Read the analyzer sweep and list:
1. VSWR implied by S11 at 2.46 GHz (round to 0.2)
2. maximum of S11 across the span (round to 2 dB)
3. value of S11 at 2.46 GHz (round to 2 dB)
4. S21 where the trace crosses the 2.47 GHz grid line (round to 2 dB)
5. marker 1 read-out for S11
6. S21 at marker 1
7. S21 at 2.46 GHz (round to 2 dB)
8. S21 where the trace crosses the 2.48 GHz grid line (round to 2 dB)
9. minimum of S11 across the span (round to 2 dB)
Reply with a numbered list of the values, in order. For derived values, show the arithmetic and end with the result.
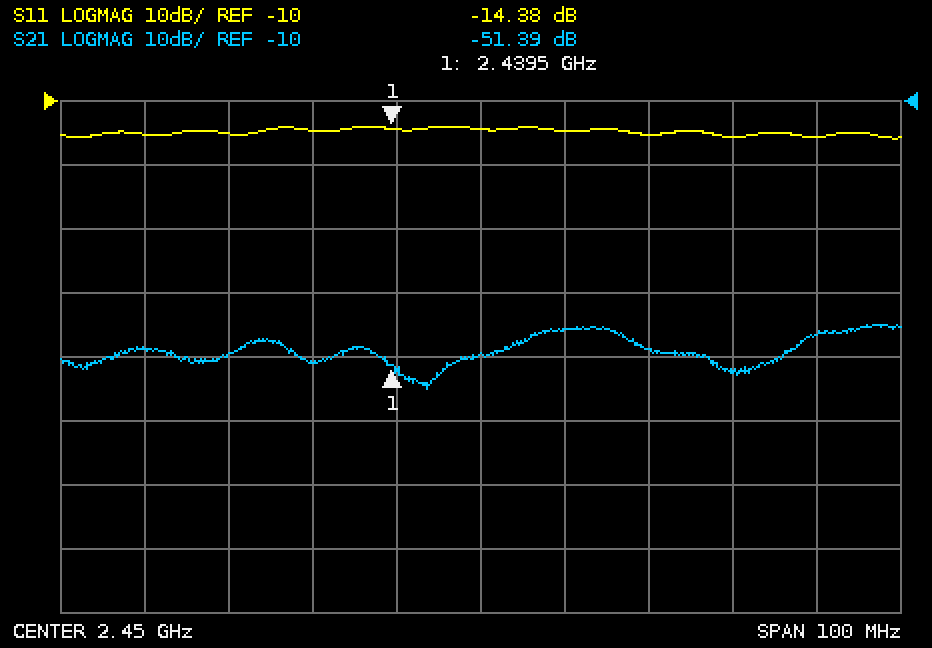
1. |Γ| = 10^(-14/20) = 0.1995; VSWR = (1 + 0.1995)/(1 − 0.1995) ≈ 1.50, so 1.4 to the nearest 0.2
2. -14 dB
3. -14 dB
4. -48 dB
5. -14.38 dB
6. -51.39 dB
7. -46 dB
8. -52 dB
9. -16 dB
